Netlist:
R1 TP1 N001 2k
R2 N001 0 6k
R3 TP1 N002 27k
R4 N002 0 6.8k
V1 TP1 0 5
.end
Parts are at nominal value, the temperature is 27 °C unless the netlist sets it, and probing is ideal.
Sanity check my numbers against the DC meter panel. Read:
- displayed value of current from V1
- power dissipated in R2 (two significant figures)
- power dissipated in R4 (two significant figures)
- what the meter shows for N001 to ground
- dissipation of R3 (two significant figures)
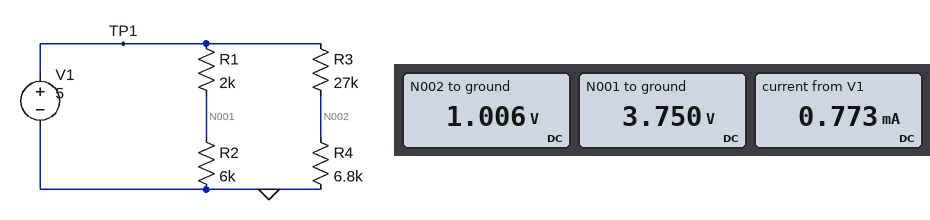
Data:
0.773 mA
2.3 mW
150 µW
3.750 V
590 µW
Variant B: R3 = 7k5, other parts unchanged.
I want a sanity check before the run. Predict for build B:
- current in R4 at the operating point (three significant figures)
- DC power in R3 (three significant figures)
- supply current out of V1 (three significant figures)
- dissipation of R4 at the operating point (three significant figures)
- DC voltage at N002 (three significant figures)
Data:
350 µA
917 µW
975 µA
831 µW
2.38 V
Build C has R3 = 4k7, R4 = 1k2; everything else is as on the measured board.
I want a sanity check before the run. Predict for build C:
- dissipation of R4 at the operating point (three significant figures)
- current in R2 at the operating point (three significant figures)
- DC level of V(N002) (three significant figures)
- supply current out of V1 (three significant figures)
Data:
862 µW
625 µA
1.02 V
1.47 mA
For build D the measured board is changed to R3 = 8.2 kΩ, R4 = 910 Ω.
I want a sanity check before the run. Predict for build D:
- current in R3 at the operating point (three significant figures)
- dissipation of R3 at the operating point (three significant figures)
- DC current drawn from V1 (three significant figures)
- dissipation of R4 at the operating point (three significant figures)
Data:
549 µA
2.47 mW
1.17 mA
274 µW
